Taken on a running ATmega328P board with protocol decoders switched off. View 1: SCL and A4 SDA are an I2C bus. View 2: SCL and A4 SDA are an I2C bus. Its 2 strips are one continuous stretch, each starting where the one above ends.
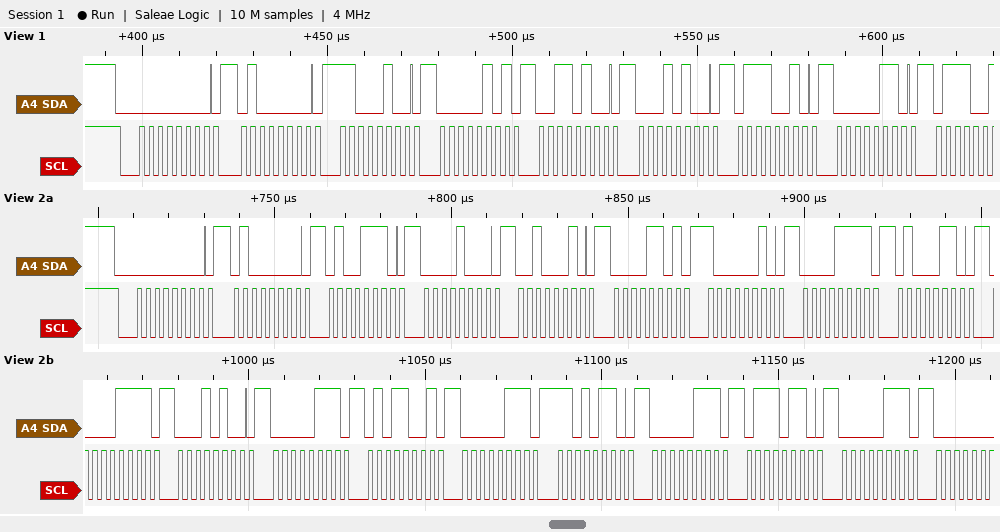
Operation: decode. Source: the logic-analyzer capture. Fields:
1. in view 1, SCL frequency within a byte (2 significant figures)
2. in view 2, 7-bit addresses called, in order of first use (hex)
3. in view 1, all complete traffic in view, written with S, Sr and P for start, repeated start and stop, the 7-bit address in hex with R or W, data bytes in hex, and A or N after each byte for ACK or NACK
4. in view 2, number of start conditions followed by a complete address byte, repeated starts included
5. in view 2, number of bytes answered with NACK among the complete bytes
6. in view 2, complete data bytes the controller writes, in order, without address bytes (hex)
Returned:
400 kHz
0x00
S 00W A 40 A C4 A 05 A 34 A 14 A 72 A 06 A
1
0
40 4E 08 22 0D 82 0F 46 0F 14 07 59 07 D6 07 76 07
